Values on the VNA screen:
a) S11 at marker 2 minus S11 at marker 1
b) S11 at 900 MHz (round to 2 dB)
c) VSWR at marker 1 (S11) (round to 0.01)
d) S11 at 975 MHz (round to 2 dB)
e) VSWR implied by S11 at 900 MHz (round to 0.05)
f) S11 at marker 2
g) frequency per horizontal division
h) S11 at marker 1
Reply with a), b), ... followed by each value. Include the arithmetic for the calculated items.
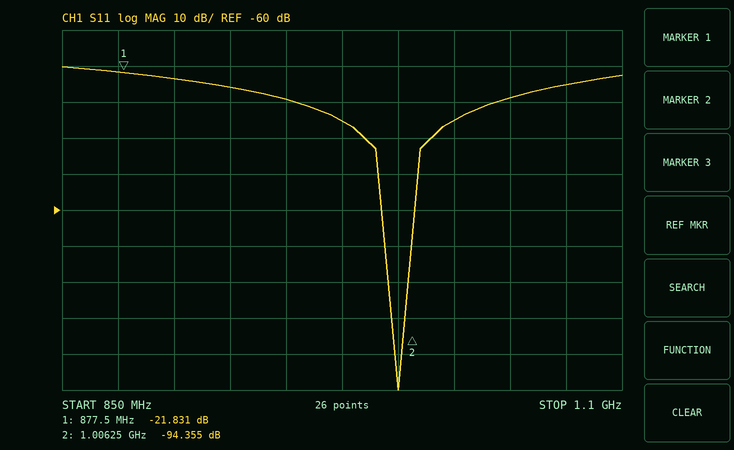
a) -94.355 − (-21.831) = -72.524 dB
b) -24 dB
c) (1 + 0.0810)/(1 − 0.0810) ≈ 1.18
d) -36 dB
e) |Γ| = 10^(-24/20) = 0.0631; VSWR = (1 + 0.0631)/(1 − 0.0631) ≈ 1.13, so 1.15 to the nearest 0.05
f) -94.355 dB
g) 25 MHz
h) -21.831 dB
